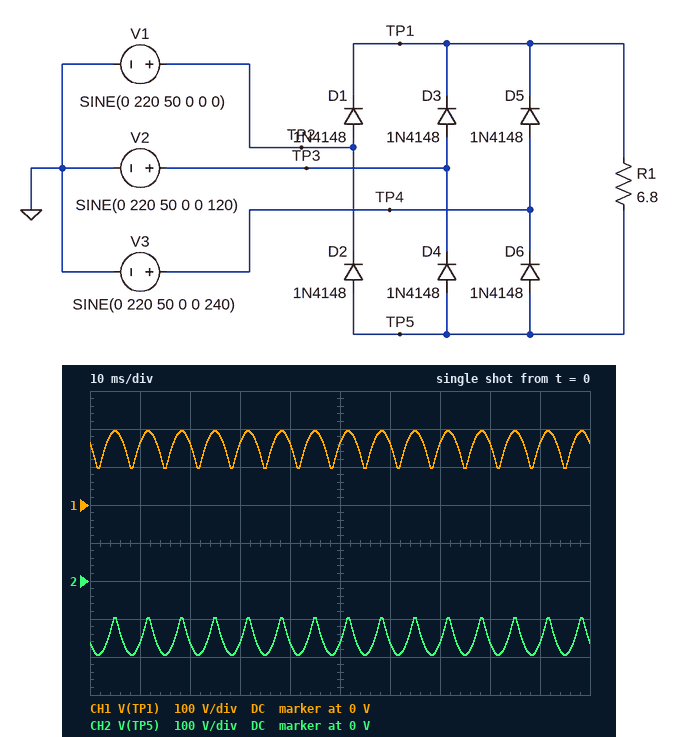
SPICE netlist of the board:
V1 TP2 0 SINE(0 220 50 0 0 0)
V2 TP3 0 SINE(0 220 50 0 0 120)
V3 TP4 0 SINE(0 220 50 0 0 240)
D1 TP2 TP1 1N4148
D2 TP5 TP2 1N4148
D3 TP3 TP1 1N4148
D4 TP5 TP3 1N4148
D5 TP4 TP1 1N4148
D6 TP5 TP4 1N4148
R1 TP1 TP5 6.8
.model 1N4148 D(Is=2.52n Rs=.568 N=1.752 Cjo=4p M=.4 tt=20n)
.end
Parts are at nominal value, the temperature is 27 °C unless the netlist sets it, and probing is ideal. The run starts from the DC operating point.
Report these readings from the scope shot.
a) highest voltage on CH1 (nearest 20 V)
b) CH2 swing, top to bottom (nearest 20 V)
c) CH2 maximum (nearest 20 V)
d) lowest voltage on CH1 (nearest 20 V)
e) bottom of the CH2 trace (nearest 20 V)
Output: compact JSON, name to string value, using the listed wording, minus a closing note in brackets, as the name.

{"highest voltage on CH1": "200 V", "CH2 swing, top to bottom": "100 V", "CH2 maximum": "-100 V", "lowest voltage on CH1": "100 V", "bottom of the CH2 trace": "-200 V"}
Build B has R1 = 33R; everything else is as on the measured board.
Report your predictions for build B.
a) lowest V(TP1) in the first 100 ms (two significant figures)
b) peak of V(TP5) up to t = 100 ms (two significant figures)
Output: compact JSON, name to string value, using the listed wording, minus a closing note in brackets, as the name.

{"lowest V(TP1) in the first 100 ms": "110 V", "peak of V(TP5) up to t = 100 ms": "-110 V"}
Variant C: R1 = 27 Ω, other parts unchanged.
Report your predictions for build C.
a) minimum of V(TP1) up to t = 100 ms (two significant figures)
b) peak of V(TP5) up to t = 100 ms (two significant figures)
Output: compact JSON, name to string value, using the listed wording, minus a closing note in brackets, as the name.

{"minimum of V(TP1) up to t = 100 ms": "110 V", "peak of V(TP5) up to t = 100 ms": "-110 V"}
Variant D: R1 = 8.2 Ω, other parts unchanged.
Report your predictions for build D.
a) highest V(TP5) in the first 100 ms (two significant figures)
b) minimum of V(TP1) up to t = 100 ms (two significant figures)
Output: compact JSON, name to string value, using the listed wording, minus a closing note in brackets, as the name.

{"highest V(TP5) in the first 100 ms": "-99 V", "minimum of V(TP1) up to t = 100 ms": "99 V"}
